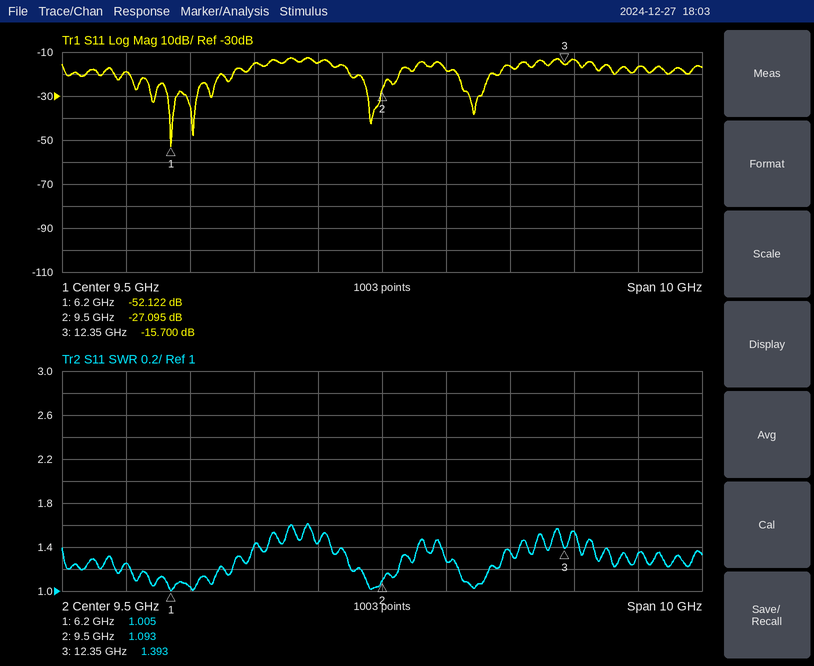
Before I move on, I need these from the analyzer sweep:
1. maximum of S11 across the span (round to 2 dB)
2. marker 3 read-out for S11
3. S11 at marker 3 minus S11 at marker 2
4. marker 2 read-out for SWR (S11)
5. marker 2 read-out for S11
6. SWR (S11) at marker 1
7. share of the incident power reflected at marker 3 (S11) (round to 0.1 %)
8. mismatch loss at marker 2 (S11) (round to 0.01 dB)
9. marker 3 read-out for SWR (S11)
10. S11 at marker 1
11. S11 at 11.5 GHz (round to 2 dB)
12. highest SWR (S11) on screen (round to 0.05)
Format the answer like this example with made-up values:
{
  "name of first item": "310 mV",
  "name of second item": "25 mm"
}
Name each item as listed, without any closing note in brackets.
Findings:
{
  "maximum of S11 across the span": "-12 dB",
  "marker 3 read-out for S11": "-15.700 dB",
  "S11 at marker 3 minus S11 at marker 2": "11.395 dB",
  "marker 2 read-out for SWR": "1.093",
  "marker 2 read-out for S11": "-27.095 dB",
  "SWR (S11) at marker 1": "1.005",
  "share of the incident power reflected at marker 3 (S11)": "2.7 %",
  "mismatch loss at marker 2 (S11)": "0.01 dB",
  "marker 3 read-out for SWR": "1.393",
  "S11 at marker 1": "-52.122 dB",
  "S11 at 11.5 GHz": "-16 dB",
  "highest SWR (S11) on screen": "1.60"
}
